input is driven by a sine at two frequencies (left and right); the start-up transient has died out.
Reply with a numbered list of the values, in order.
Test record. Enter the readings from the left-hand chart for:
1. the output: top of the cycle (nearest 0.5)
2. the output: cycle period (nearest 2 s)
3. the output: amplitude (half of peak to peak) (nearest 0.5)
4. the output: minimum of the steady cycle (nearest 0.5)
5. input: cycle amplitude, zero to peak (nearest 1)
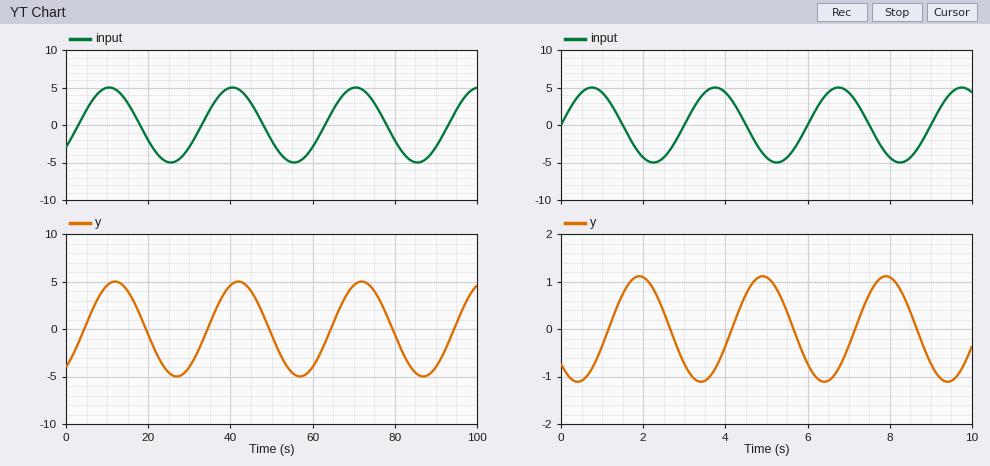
1. 5.0
2. 30 s
3. 5.0
4. -5.0
5. 5
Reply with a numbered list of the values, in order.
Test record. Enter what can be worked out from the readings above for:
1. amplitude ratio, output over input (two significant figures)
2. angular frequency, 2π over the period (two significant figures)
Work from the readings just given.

1. 1.0
2. 0.21 rad/s
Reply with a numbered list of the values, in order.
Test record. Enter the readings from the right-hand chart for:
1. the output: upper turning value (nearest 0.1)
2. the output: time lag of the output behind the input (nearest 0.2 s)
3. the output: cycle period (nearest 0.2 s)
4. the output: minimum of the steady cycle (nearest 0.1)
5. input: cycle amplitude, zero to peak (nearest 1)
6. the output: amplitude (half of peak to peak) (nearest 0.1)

1. 1.1
2. 1.2 s
3. 3.0 s
4. -1.1
5. 5
6. 1.1
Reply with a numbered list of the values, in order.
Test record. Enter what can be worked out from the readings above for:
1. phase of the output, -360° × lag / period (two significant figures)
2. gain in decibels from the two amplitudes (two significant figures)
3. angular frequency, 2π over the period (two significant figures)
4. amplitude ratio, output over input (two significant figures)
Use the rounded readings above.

1. -140°
2. -13 dB
3. 2.1 rad/s
4. 0.22
